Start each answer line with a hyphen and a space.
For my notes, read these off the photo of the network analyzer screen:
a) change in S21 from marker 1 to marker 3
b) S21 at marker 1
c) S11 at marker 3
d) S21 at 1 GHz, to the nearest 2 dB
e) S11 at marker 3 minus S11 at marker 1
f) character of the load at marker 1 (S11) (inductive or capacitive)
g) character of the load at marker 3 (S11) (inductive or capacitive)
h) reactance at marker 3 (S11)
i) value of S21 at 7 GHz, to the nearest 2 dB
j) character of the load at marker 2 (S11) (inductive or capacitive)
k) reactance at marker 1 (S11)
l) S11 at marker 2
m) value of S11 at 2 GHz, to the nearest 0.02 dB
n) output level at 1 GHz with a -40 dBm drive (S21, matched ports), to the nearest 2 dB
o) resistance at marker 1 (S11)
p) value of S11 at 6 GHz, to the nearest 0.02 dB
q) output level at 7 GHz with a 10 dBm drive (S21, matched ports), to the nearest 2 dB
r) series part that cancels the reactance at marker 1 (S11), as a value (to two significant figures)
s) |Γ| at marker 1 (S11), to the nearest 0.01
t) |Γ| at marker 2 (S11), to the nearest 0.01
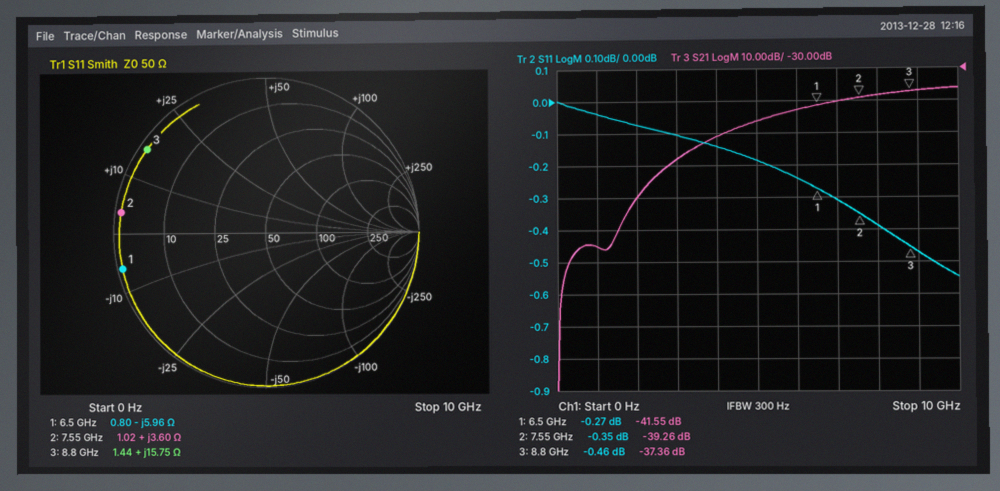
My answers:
- 4.19 dB
- -41.55 dB
- -0.46 dB
- -86 dB
- -0.19 dB
- capacitive
- inductive
- +15.75 Ω
- -40 dB
- inductive
- -5.96 Ω
- -0.35 dB
- -0.08 dB
- -126 dBm
- 0.80 Ω
- -0.24 dB
- -30 dBm
- 150 pH
- 0.97
- 0.96
